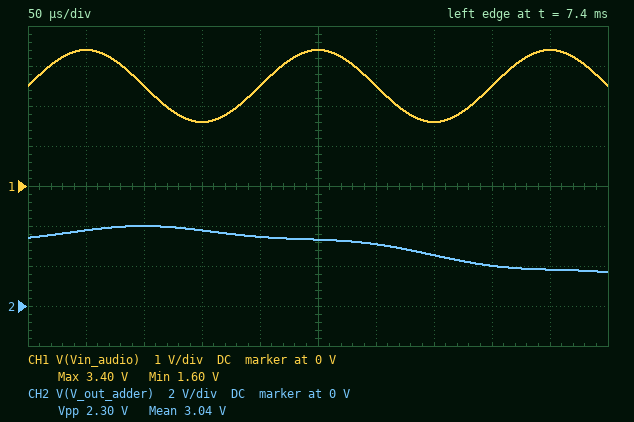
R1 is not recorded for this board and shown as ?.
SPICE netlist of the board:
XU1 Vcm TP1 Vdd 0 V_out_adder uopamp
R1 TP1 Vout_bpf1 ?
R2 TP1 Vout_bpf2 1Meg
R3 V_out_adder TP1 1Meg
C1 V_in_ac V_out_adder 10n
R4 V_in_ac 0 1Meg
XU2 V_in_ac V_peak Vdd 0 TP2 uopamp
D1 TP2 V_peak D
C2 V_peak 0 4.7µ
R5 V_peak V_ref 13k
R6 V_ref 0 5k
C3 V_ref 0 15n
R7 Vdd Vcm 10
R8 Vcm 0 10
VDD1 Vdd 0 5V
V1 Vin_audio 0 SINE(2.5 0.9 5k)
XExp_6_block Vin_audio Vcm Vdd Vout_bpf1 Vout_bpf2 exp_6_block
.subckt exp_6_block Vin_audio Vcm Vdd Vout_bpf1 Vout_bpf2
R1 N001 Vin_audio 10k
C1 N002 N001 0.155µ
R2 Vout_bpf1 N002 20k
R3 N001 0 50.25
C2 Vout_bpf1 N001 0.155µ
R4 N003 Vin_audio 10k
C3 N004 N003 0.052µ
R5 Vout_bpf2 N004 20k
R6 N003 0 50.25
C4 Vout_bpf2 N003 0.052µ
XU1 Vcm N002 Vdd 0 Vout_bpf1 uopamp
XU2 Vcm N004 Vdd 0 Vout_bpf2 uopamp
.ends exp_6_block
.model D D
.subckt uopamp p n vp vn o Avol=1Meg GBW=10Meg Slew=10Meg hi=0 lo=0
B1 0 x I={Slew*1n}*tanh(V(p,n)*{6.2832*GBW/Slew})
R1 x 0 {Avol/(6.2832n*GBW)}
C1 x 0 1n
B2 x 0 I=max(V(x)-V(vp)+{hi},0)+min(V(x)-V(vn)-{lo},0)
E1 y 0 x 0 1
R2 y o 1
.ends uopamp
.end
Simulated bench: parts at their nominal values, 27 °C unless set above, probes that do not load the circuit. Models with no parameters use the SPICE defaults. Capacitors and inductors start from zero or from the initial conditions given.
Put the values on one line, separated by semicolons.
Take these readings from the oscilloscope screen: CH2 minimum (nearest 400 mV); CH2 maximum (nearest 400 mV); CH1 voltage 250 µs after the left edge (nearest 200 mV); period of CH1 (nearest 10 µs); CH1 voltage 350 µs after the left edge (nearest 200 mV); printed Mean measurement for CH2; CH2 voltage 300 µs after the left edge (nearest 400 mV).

1.6 V; 4.0 V; 3.4 V; 200 µs; 1.6 V; 3.04 V; 3.2 V
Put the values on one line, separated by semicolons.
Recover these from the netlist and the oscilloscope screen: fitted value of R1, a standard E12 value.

330 kΩ
